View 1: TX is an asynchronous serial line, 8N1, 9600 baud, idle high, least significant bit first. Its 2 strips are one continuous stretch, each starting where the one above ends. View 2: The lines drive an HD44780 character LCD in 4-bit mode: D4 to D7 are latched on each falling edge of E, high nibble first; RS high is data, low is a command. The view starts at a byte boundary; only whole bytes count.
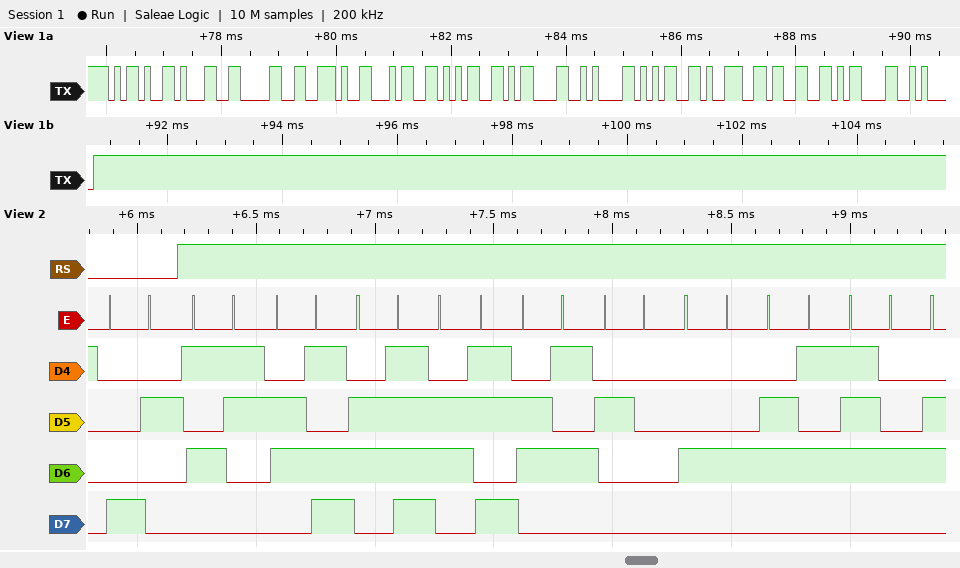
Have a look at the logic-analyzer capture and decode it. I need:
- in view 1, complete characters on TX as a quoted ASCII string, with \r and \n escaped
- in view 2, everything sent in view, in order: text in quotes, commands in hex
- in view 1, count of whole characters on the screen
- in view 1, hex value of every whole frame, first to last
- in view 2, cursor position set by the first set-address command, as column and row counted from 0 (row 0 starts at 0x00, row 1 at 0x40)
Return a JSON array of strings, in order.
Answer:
["\"-10.45\\r\\n593\\r\\n\"", "0x82 \"Smoke Det\"", "13", "2D 31 30 2E 34 35 0D 0A 35 39 33 0D 0A", "column 2, row 0"]
